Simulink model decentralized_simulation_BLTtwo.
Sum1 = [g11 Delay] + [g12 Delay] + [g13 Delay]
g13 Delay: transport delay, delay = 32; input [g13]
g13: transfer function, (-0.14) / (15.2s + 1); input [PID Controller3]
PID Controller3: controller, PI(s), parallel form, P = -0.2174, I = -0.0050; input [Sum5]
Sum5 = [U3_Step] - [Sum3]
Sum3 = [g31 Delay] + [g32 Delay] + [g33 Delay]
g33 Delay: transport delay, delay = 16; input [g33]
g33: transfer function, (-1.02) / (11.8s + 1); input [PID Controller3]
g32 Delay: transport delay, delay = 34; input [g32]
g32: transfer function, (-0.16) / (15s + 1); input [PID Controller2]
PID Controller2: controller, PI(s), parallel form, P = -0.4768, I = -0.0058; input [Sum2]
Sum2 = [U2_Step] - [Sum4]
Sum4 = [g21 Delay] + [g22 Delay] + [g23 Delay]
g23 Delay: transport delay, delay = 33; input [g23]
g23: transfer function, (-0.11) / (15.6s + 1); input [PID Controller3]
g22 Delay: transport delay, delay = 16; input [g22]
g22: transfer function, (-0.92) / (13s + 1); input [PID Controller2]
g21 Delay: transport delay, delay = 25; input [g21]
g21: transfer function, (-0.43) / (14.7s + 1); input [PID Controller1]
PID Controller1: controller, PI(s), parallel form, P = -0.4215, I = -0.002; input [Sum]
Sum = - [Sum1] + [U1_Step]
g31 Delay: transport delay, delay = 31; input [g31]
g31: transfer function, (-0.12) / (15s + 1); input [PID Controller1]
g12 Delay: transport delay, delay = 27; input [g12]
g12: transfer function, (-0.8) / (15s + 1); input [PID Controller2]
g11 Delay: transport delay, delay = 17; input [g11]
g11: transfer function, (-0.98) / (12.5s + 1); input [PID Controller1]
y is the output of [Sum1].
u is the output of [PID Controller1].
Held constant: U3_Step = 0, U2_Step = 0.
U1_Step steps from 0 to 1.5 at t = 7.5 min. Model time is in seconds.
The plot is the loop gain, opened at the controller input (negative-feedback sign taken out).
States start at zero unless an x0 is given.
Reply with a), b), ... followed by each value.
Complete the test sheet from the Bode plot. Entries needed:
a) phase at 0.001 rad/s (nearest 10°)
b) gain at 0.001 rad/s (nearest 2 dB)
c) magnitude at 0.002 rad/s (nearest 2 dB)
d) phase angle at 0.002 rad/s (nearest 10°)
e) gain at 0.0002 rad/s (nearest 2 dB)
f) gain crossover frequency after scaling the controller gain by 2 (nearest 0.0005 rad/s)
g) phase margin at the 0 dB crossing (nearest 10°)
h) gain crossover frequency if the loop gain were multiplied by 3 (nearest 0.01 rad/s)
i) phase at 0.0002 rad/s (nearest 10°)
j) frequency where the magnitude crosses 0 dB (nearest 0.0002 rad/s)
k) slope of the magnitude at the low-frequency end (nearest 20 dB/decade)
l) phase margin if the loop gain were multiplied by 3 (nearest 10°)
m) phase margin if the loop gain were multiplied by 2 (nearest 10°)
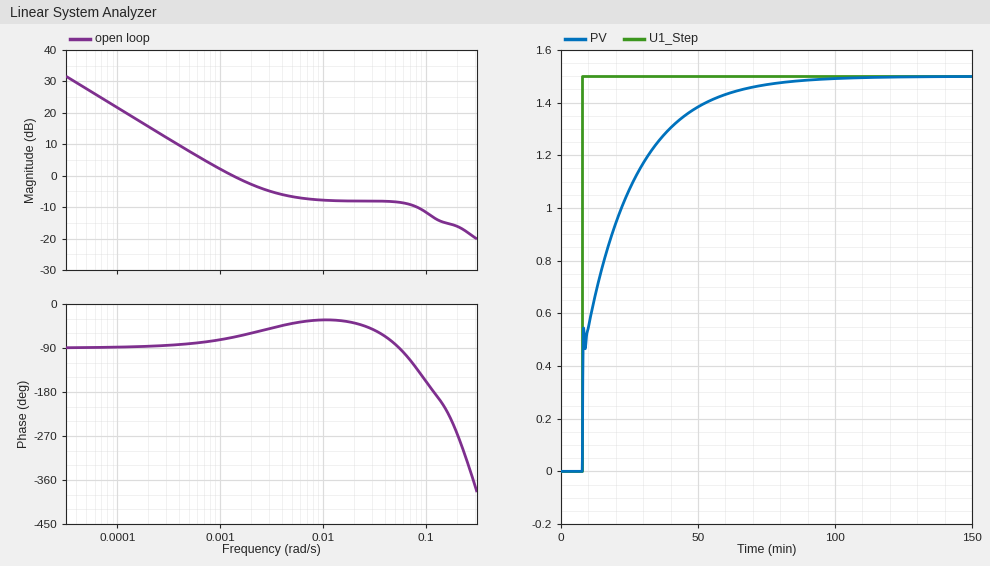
a) -70°
b) 2 dB
c) -2 dB
d) -60°
e) 16 dB
f) 0.0040 rad/s
g) 110°
h) 0.08 rad/s
i) -90°
j) 0.0014 rad/s
k) -20 dB/decade
l) 60°
m) 140°
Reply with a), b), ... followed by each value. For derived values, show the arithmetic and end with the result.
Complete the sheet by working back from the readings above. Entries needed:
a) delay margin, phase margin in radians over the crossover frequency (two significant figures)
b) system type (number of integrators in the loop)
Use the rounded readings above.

a) 110 × π / 180 / 0.0014 = 1400 s
b) 1
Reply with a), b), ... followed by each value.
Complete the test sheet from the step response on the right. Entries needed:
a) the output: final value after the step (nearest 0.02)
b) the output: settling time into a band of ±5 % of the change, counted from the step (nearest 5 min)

a) 1.50
b) 50 min
